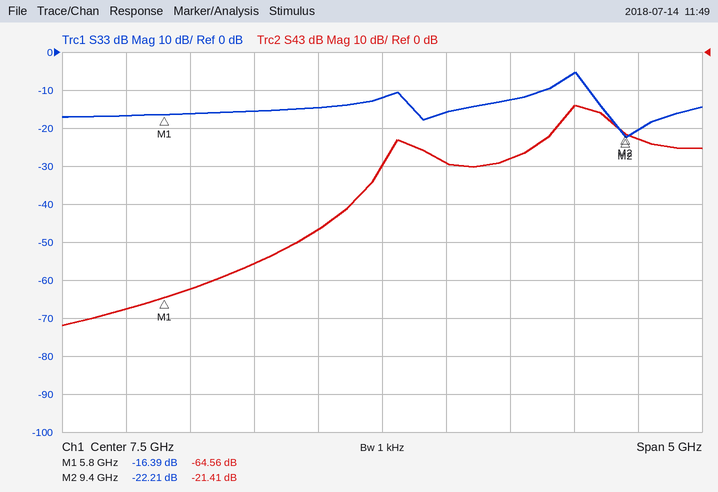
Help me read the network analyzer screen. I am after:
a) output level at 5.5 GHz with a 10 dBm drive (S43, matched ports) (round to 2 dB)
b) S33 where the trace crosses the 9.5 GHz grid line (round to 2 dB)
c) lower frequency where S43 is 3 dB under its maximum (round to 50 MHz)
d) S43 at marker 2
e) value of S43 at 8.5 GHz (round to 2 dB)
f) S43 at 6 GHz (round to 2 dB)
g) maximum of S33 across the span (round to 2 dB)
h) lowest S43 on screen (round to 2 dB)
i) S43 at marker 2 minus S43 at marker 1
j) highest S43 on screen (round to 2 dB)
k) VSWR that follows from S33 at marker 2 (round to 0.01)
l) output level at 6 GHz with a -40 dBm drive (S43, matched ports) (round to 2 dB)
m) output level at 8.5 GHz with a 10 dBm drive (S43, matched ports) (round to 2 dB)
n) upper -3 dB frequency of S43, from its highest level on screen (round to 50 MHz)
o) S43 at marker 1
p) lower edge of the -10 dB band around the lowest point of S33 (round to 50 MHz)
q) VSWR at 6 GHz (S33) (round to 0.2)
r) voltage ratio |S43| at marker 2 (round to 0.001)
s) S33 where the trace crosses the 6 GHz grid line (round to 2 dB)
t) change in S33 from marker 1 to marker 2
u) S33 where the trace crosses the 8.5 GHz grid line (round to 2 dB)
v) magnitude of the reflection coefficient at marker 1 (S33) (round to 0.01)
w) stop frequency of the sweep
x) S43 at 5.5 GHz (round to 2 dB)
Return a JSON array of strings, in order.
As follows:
["-58 dBm", "-20 dB", "8.95 GHz", "-21.41 dB", "-28 dB", "-62 dB", "-6 dB", "-72 dB", "43.15 dB", "-14 dB", "1.17", "-102 dBm", "-18 dBm", "9.25 GHz", "-64.56 dB", "9.10 GHz", "1.4", "0.085", "-16 dB", "-5.82 dB", "-12 dB", "0.15", "10 GHz", "-68 dB"]
